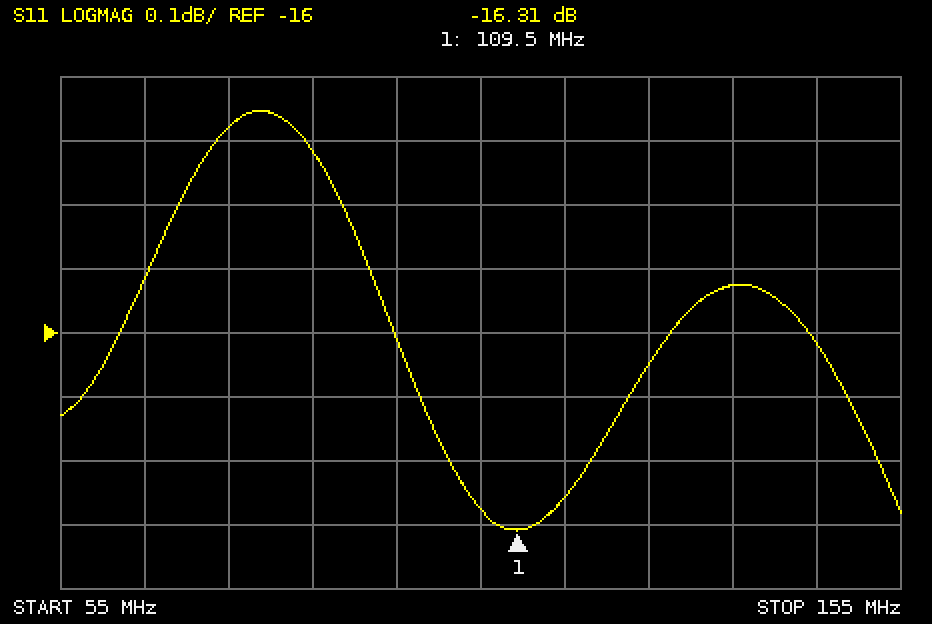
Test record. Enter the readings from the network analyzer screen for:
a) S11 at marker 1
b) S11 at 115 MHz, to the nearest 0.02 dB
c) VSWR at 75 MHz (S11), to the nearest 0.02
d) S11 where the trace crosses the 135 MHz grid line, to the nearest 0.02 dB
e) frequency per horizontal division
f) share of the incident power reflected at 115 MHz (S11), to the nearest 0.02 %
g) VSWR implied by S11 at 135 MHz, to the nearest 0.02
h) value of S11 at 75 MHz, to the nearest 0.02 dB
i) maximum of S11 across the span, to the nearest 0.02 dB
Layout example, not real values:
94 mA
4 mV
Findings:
-16.31 dB
-16.26 dB
1.40
-15.92 dB
10 MHz
2.36 %
1.38
-15.68 dB
-15.66 dB
